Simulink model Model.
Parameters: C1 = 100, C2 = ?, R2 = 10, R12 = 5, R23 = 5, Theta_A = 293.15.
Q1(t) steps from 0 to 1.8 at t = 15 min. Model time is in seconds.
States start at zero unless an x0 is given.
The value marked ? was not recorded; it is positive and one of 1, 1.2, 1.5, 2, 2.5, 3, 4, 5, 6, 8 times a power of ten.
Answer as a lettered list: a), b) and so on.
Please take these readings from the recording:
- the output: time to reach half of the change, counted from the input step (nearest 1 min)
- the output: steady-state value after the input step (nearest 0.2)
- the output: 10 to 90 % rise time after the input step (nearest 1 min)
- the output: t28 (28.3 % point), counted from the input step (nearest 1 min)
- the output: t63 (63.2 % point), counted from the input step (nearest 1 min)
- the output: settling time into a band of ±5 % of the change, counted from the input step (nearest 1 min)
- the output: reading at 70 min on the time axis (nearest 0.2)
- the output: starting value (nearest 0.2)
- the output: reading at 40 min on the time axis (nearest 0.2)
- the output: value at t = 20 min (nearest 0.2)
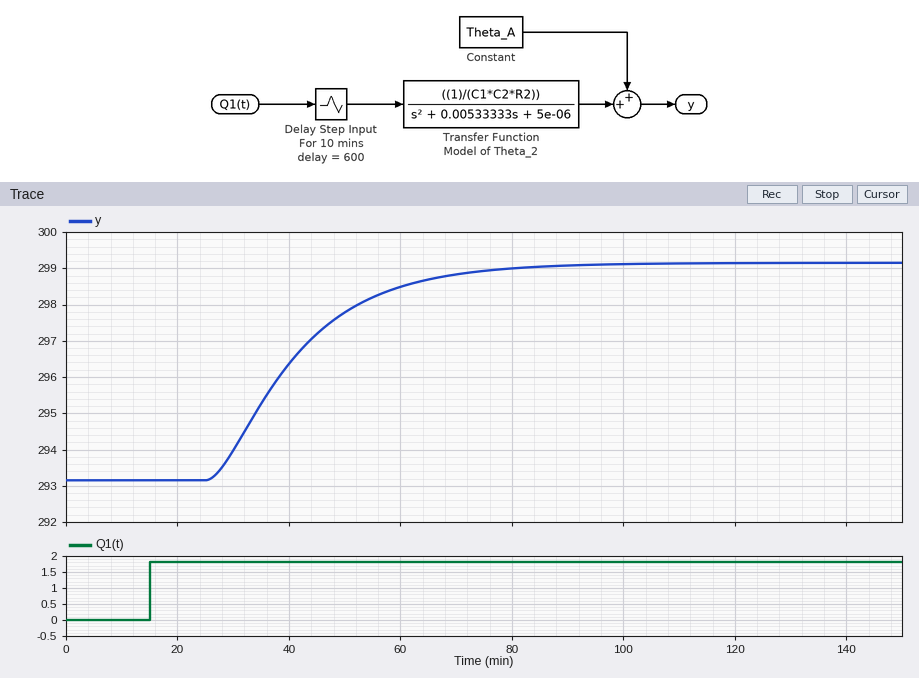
a) 24 min
b) 299.2
c) 32 min
d) 18 min
e) 28 min
f) 56 min
g) 298.8
h) 293.2
i) 296.4
j) 293.2
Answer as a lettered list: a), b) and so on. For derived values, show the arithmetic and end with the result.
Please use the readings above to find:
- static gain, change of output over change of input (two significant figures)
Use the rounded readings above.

a) (299.2 - 293.2) / (1.8 - 0) = 3.3
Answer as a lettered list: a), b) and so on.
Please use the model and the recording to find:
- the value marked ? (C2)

a) 60
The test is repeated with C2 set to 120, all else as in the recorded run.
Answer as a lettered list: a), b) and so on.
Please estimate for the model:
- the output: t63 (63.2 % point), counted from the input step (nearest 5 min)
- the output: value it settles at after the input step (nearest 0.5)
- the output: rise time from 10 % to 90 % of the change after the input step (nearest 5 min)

a) 35 min
b) 299.0
c) 45 min
